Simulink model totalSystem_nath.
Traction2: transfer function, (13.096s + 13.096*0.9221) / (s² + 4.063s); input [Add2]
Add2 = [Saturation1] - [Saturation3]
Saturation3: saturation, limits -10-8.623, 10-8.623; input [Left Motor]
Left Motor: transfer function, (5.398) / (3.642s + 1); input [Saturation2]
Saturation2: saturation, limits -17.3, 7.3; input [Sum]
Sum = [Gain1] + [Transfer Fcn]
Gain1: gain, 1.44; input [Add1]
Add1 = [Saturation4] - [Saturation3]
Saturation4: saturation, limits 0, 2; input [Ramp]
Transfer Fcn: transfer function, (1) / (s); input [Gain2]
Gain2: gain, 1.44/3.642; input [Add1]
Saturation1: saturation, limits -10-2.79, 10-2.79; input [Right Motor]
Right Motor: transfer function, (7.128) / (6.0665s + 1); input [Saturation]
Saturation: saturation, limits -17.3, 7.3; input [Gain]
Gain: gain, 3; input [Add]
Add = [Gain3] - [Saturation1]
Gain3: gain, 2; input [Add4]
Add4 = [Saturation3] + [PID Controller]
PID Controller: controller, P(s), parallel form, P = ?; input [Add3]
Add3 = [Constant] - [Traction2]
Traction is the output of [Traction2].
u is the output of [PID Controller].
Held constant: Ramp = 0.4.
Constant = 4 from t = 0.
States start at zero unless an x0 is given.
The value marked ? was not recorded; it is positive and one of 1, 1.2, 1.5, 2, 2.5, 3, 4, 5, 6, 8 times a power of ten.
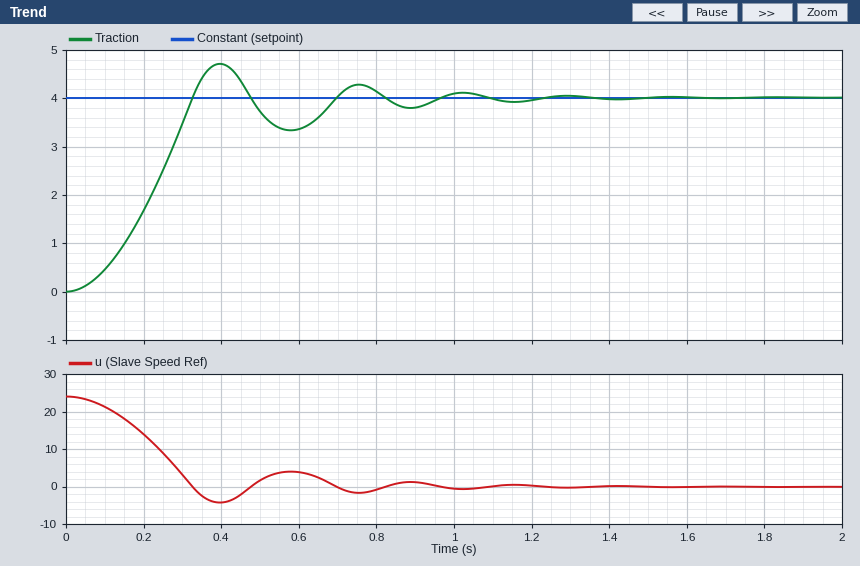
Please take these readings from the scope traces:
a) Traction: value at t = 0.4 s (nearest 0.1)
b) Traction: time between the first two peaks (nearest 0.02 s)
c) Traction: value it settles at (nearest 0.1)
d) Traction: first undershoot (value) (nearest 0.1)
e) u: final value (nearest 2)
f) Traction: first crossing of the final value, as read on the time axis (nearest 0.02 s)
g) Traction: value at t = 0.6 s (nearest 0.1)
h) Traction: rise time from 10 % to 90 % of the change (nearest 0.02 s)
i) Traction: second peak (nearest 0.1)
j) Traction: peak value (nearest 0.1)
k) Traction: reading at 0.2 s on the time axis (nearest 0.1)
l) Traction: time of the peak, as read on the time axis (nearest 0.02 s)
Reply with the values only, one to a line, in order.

4.7
0.36 s
4.0
3.3
0
0.32 s
3.4
0.22 s
4.3
4.7
1.7
0.40 s
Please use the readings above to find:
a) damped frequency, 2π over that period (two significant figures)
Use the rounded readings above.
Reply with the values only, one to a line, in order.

17 rad/s
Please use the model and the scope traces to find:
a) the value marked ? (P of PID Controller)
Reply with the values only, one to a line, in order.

6
